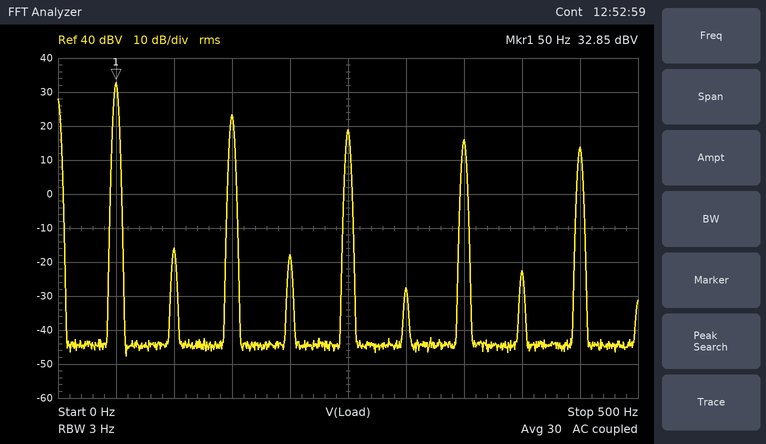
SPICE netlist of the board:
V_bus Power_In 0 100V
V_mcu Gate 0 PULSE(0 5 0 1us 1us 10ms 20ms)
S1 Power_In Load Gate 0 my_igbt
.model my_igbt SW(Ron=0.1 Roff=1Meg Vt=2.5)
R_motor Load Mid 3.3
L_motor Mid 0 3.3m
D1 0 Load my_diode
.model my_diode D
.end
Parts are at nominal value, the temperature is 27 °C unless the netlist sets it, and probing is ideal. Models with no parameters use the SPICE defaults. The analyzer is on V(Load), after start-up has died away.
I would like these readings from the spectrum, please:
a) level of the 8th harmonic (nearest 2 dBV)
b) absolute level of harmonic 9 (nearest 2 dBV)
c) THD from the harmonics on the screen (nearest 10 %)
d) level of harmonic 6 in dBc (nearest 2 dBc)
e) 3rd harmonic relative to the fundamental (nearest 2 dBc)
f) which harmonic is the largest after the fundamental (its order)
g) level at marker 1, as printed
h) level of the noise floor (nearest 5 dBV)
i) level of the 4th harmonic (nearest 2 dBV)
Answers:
-22 dBV
14 dBV
40 %
-60 dBc
-10 dBc
3
32.85 dBV
-45 dBV
-18 dBV
